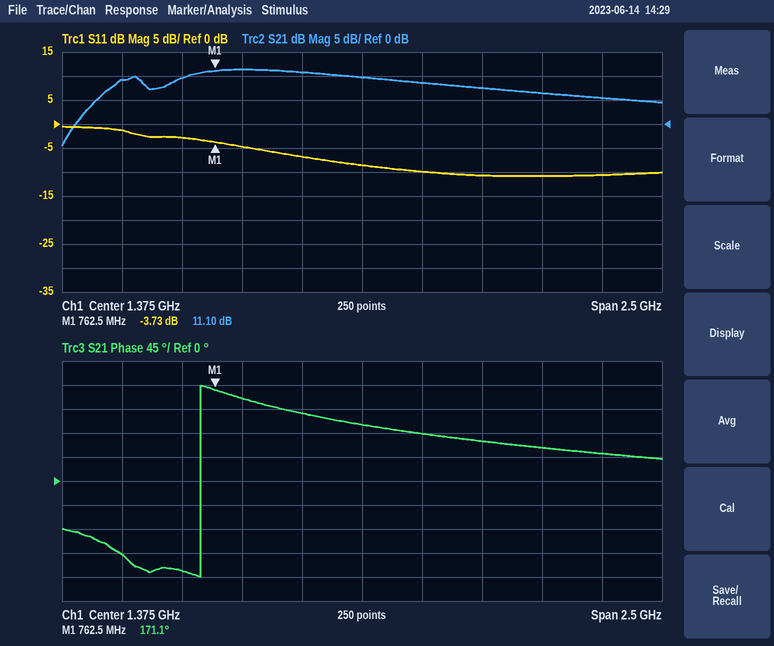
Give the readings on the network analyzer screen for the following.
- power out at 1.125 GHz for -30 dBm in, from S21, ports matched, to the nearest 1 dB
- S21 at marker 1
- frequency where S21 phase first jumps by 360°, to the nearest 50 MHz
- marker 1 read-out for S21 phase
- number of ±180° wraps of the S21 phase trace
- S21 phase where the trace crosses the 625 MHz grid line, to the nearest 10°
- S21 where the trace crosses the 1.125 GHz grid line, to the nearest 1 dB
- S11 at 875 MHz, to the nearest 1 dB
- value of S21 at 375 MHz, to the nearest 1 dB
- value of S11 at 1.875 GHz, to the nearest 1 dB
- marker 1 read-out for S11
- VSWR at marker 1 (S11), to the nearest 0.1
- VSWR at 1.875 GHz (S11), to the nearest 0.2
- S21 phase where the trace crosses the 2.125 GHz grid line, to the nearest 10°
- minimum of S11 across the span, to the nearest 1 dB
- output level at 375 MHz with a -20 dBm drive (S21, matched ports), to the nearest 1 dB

-19 dBm
11.10 dB
700 MHz
171.1°
1
-170°
11 dB
-5 dB
9 dB
-11 dB
-3.73 dB
4.7
1.8
60°
-11 dB
-11 dBm
